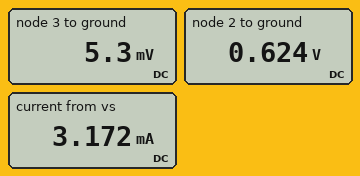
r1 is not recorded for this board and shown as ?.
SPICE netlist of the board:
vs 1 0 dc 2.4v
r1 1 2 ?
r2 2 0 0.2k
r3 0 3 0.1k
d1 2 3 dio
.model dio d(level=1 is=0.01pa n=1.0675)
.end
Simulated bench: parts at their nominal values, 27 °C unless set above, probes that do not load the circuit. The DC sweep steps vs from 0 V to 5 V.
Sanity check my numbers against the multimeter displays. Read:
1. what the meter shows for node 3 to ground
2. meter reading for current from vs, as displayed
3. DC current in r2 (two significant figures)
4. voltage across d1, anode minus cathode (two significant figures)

5.3 mV
3.172 mA
3.1 mA
620 mV
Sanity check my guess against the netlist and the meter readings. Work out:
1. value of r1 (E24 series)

560 Ω
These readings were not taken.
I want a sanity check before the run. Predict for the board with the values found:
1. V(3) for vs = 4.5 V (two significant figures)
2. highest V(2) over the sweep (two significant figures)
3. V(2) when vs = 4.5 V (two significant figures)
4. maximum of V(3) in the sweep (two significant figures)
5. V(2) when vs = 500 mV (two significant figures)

190 mV
960 mV
910 mV
240 mV
130 mV
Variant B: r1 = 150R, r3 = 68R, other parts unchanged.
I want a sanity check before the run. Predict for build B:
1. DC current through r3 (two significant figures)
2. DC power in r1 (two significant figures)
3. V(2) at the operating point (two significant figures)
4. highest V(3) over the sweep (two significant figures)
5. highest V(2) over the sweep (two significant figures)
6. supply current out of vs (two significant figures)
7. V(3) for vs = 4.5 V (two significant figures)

4.1 mA
13 mW
1.0 V
920 mV
1.7 V
9.2 mA
800 mV
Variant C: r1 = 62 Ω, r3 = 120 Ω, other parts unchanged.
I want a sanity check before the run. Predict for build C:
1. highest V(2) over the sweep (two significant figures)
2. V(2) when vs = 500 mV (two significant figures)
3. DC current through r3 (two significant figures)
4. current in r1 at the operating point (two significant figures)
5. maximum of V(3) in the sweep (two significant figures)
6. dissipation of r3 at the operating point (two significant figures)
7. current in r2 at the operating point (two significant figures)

3.0 V
380 mV
6.5 mA
14 mA
2.2 V
5.0 mW
7.6 mA
